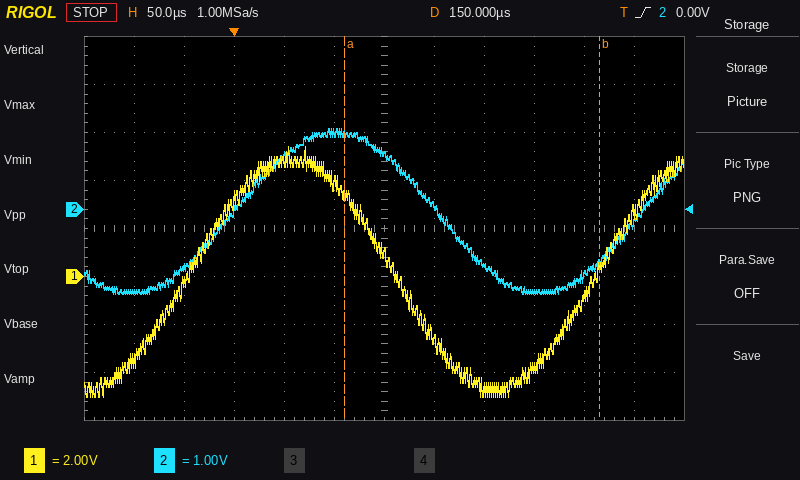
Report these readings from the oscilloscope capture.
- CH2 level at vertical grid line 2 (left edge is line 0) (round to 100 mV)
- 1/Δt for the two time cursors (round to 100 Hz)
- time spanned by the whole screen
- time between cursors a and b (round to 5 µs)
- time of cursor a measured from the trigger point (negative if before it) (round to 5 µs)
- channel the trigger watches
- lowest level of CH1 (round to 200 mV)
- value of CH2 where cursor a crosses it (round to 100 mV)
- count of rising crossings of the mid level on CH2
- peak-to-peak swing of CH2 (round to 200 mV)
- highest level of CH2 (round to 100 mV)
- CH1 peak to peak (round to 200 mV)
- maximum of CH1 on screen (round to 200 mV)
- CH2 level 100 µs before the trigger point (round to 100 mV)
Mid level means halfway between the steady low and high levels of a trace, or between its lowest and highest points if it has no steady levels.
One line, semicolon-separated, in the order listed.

-1.2 V; 3.9 kHz; 600 µs; 255 µs; +110 µs; CH2; -5.0 V; 1.6 V; 2; 3.4 V; 1.7 V; 10.4 V; 5.4 V; -1.7 V
